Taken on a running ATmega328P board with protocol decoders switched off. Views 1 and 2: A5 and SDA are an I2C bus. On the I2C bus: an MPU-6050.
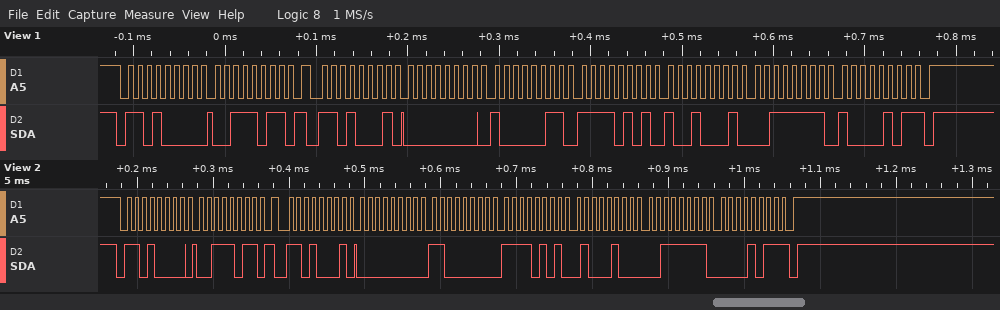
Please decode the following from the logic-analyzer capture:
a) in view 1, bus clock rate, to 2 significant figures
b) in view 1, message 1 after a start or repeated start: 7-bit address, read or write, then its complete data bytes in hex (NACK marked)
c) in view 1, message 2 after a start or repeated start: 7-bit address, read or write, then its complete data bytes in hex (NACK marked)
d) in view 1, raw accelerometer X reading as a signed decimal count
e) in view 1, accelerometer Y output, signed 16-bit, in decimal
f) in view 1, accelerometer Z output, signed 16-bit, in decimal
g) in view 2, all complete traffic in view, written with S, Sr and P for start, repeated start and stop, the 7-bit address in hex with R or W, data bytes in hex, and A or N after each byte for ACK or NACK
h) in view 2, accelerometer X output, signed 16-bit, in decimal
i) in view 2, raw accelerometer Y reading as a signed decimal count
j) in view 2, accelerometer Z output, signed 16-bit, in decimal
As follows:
100 kHz
0x68 write: 3B
0x68 read: 00 83 F5 91 3F 85 NACK
131
-2671
16261
S 68W A 3B A Sr 68R A 00 A C0 A F5 A 44 A 3F A 0B N P
192
-2748
16139
